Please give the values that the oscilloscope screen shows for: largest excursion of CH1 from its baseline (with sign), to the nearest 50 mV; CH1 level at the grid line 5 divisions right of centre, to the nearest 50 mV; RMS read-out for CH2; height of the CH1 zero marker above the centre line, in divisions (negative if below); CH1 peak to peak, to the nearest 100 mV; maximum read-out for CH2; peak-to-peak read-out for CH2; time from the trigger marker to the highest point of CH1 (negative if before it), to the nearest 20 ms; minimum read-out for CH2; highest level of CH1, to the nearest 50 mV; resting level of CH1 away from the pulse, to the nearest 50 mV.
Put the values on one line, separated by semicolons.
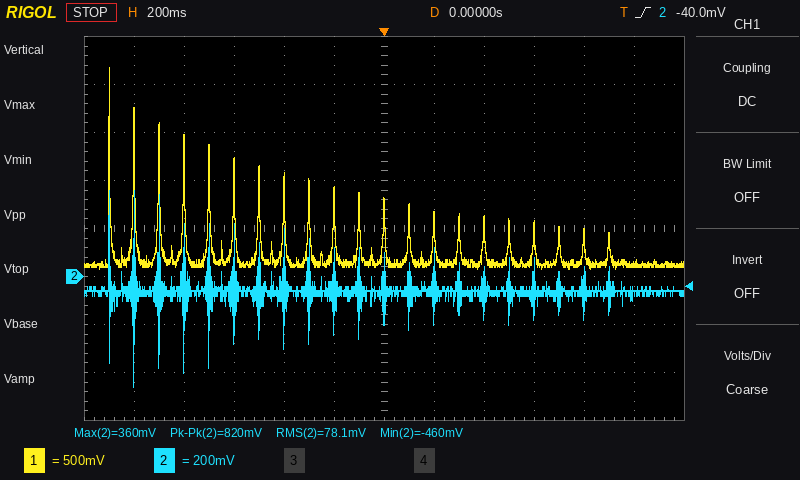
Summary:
+2.05 V; 150 mV; 78.1 mV; -1.0 div; 2.10 V; 360 mV; 820 mV; -1.10 s; -460 mV; 2.20 V; 150 mV
